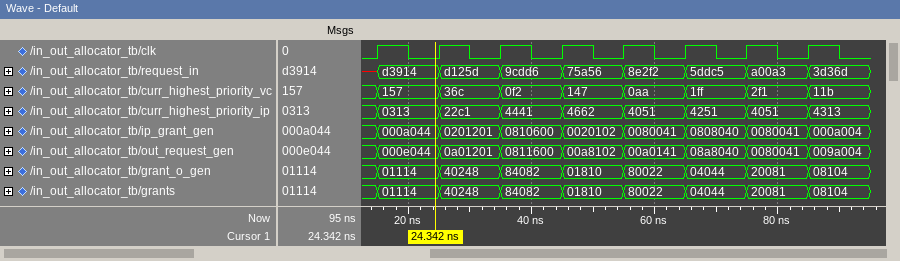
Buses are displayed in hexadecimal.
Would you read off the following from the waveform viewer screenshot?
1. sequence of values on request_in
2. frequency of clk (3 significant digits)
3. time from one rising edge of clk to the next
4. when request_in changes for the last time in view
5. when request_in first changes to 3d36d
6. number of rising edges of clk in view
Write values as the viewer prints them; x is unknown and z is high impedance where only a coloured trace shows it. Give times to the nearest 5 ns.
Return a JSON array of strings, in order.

["x, d3914, d125d, 9cdd6, 75a56, 8e2f2, 5ddc5, a00a3, 3d36d", "100 MHz", "10 ns", "85 ns", "85 ns", "8"]
